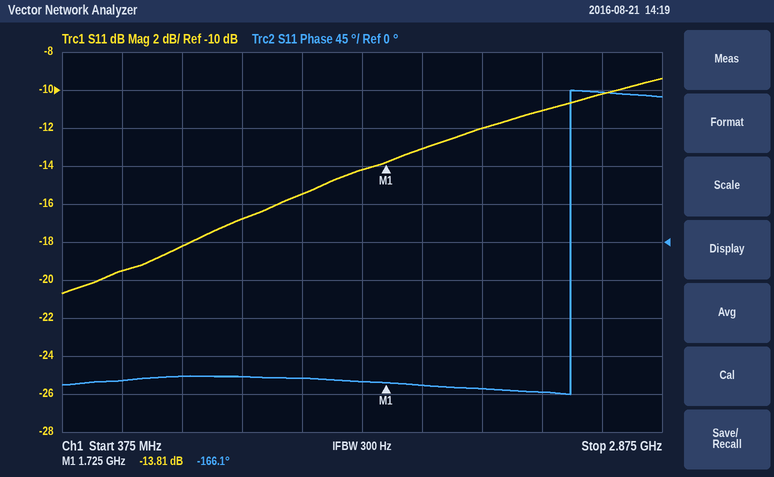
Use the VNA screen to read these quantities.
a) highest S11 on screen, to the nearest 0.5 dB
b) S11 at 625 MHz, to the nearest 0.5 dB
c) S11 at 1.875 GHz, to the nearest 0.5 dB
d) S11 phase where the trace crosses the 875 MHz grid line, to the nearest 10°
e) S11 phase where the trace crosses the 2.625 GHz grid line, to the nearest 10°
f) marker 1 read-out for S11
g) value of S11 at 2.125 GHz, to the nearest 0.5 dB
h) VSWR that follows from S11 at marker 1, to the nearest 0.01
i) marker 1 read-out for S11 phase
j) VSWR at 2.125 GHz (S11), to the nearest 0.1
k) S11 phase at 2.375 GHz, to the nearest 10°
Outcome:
-9.5 dB
-19.5 dB
-13.0 dB
-160°
180°
-13.81 dB
-12.0 dB
1.51
-166.1°
1.7
-180°
